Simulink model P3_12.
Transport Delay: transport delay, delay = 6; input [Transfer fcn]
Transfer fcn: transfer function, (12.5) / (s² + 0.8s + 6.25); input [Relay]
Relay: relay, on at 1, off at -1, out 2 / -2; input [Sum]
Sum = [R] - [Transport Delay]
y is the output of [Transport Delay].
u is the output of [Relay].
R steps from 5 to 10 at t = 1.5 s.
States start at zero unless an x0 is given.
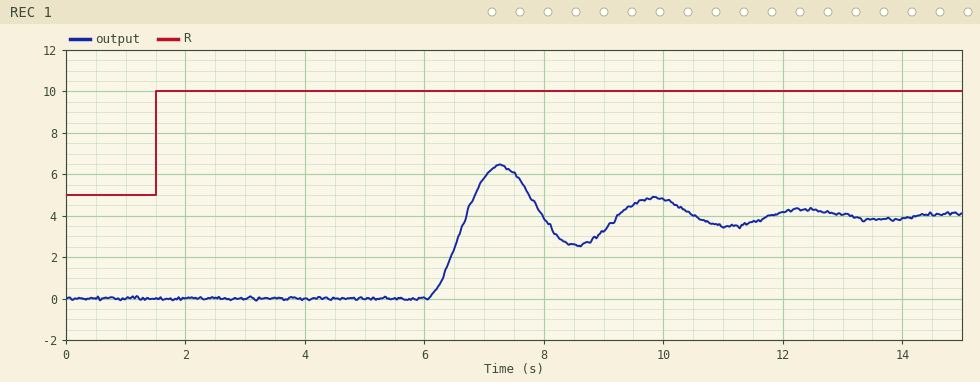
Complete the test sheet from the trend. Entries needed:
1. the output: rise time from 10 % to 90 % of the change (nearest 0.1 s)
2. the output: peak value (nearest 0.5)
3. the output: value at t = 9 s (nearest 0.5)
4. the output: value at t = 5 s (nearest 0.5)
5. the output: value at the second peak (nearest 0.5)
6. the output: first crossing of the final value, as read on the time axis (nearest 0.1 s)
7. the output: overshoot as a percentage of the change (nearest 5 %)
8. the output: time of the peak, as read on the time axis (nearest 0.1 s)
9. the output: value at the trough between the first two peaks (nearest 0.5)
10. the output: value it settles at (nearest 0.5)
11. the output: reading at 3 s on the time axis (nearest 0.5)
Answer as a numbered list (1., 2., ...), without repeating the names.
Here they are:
1. 0.5 s
2. 6.5
3. 3.5
4. 0.0
5. 5.0
6. 6.7 s
7. 60 %
8. 7.3 s
9. 2.5
10. 4.0
11. 0.0
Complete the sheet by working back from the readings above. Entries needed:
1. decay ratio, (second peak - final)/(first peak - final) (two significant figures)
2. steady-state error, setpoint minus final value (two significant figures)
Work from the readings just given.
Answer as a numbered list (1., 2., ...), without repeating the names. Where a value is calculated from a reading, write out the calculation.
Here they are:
1. (5 - 4) / (6.5 - 4) = 0.40
2. 10 - 4 = 6.0
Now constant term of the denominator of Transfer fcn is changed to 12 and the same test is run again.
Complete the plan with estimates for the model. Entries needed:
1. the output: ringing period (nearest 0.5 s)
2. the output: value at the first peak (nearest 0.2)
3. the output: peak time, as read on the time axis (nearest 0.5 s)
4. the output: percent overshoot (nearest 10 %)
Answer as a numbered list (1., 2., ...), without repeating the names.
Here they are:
1. 2.0 s
2. 3.6
3. 7.0 s
4. 70 %
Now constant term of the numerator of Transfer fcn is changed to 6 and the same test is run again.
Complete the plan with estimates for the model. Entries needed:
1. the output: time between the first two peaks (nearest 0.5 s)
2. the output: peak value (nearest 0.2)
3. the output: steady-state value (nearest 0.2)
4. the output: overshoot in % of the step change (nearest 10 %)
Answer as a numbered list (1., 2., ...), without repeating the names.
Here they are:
1. 2.5 s
2. 3.0
3. 2.0
4. 60 %
